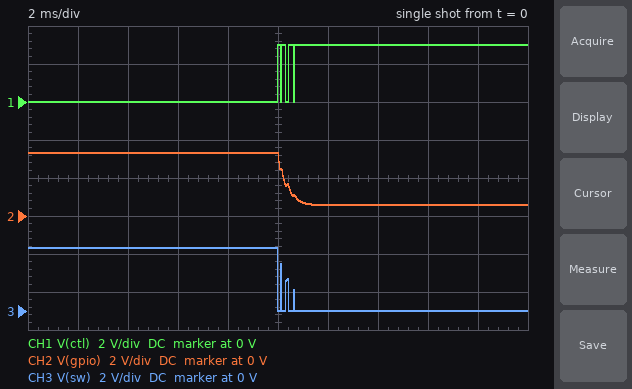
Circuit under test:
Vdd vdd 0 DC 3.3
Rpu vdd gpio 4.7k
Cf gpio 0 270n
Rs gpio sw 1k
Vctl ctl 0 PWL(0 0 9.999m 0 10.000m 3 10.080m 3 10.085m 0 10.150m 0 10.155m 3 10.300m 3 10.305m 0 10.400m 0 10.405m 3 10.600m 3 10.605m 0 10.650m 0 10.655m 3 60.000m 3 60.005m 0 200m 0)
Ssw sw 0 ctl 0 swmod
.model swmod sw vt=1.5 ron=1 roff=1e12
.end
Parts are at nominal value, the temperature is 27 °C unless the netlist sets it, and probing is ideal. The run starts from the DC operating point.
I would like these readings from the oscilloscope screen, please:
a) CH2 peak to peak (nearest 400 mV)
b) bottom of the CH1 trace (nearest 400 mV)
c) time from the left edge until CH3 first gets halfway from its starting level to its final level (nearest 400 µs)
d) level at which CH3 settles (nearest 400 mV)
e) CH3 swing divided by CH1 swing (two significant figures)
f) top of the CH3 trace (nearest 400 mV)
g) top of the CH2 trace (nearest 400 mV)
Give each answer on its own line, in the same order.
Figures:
2.8 V
0 V
10.0 ms
0 V
1.1
3.2 V
3.2 V
